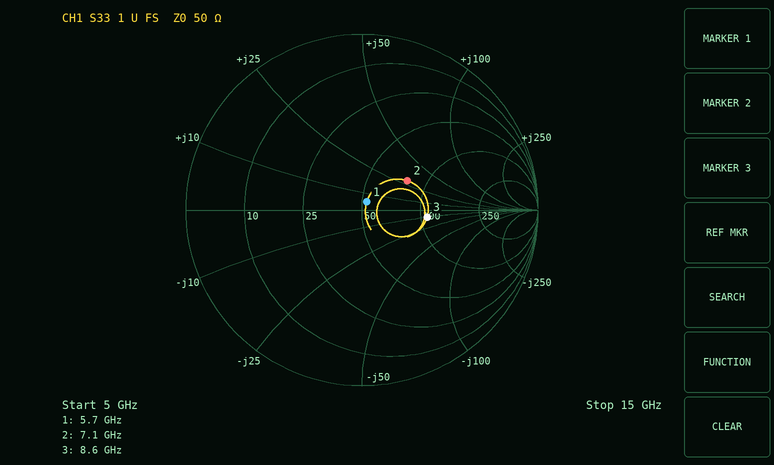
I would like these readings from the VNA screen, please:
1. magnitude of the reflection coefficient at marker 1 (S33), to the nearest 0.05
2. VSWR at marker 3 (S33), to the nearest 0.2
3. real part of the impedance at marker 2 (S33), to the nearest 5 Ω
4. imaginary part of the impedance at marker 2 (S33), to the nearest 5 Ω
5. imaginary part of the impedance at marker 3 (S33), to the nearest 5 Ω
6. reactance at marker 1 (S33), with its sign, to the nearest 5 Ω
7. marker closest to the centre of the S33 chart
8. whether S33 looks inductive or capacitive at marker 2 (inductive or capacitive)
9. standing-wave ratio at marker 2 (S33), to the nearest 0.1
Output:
0.05
2.2
80 Ω
+30 Ω
-10 Ω
+5 Ω
marker 1
inductive
1.9
